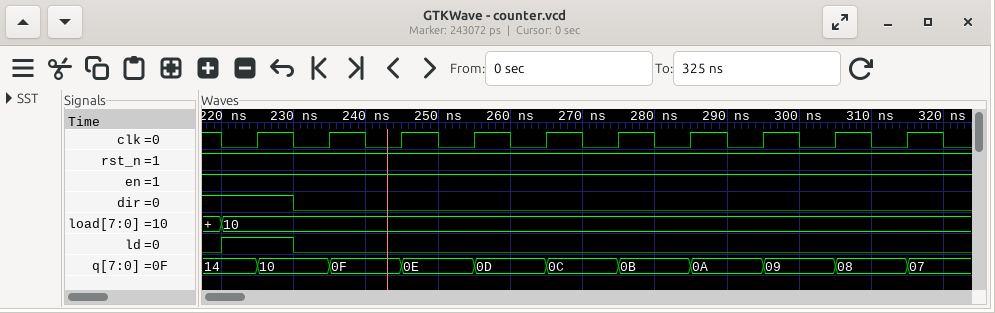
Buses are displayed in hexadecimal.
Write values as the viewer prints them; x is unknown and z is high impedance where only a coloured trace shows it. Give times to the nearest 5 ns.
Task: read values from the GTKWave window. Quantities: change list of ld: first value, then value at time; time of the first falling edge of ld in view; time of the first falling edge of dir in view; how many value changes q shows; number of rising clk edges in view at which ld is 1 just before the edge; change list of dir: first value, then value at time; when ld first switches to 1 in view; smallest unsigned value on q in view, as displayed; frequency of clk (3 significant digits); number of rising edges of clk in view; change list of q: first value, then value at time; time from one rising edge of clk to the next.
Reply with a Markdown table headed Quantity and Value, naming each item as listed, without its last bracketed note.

| Quantity | Value |
|---|---|
| change list of ld: first value, then value at time | 0, 1 at 220 ns, 0 at 230 ns |
| time of the first falling edge of ld in view | 230 ns |
| time of the first falling edge of dir in view | 230 ns |
| how many value changes q shows | 10 |
| number of rising clk edges in view at which ld is 1 just before the edge | 1 |
| change list of dir: first value, then value at time | 1, 0 at 230 ns |
| when ld first switches to 1 in view | 220 ns |
| smallest unsigned value on q in view, as displayed | 07 |
| frequency of clk | 100 MHz |
| number of rising edges of clk in view | 10 |
| change list of q: first value, then value at time | 14, 10 at 225 ns, 0F at 235 ns, 0E at 245 ns, 0D at 255 ns, 0C at 265 ns, 0B at 275 ns, 0A at 285 ns, 09 at 295 ns, 08 at 305 ns, 07 at 315 ns |
| time from one rising edge of clk to the next | 10 ns |
